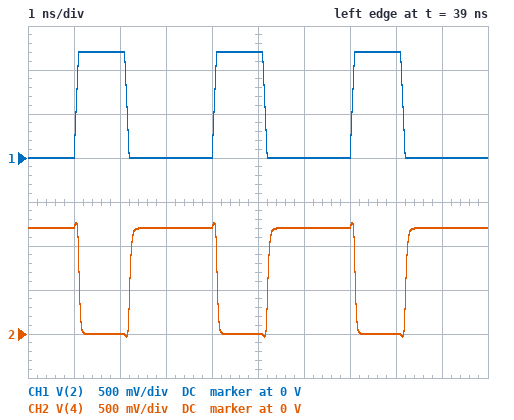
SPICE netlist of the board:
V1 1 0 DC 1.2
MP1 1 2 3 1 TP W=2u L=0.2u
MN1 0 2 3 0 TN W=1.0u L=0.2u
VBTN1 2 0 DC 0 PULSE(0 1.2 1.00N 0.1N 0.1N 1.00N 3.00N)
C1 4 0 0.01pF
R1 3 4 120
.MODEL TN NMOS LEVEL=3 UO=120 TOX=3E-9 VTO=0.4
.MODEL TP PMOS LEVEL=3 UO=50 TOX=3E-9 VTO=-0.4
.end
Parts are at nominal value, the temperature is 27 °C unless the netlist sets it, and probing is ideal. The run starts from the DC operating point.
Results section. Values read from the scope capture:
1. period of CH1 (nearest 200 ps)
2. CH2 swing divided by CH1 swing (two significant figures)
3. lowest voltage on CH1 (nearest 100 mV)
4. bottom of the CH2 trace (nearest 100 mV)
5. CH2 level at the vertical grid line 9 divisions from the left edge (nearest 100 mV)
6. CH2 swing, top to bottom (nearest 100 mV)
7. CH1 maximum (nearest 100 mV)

3.0 ns
1.1
0 V
0 V
1.2 V
1.3 V
1.2 V
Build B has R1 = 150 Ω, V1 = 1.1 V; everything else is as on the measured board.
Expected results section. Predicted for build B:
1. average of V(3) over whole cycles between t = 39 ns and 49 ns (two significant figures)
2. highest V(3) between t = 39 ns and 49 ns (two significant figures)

690 mV
1.2 V
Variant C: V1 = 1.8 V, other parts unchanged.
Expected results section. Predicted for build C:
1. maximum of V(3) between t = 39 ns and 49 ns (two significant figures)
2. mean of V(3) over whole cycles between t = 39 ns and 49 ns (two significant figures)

1.8 V
1.2 V
